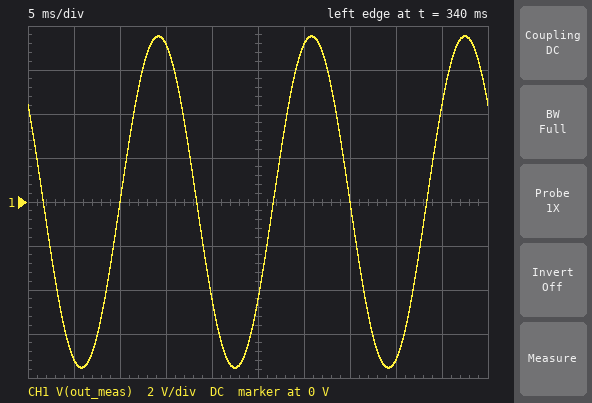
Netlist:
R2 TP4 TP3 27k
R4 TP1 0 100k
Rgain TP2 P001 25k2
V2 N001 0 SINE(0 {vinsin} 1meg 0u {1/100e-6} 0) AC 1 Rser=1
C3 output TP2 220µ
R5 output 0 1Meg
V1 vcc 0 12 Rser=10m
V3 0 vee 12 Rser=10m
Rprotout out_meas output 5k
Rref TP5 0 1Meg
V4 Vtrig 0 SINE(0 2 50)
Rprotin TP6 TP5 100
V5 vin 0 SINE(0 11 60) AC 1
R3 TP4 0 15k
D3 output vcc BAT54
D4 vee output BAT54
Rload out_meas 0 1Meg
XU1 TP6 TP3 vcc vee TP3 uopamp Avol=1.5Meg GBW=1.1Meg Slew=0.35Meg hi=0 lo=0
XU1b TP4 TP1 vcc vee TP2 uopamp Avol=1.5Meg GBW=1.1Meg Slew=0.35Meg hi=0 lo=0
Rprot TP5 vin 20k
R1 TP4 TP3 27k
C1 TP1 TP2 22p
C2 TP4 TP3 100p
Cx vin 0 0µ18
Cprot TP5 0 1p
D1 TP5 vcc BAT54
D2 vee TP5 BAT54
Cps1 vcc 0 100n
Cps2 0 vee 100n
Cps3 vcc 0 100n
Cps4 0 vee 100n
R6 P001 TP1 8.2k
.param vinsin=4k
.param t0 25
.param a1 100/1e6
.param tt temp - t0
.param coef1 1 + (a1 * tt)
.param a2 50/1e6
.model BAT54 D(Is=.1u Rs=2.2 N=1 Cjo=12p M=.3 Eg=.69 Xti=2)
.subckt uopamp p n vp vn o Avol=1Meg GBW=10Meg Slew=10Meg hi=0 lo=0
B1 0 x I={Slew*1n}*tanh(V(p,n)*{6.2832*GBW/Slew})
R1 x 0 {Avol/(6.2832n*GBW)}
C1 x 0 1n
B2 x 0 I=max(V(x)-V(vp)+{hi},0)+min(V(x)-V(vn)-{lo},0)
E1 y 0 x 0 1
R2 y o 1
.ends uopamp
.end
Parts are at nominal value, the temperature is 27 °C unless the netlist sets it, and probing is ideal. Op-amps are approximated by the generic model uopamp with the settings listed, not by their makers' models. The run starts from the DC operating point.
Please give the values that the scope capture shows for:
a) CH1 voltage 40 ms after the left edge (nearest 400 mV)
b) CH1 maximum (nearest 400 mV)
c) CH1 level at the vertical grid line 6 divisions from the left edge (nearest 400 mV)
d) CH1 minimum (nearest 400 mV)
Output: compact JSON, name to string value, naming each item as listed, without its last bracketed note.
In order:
{"CH1 voltage 40 ms after the left edge": "-7.2 V", "CH1 maximum": "7.6 V", "CH1 level at the vertical grid line 6 divisions from the left edge": "7.2 V", "CH1 minimum": "-7.6 V"}
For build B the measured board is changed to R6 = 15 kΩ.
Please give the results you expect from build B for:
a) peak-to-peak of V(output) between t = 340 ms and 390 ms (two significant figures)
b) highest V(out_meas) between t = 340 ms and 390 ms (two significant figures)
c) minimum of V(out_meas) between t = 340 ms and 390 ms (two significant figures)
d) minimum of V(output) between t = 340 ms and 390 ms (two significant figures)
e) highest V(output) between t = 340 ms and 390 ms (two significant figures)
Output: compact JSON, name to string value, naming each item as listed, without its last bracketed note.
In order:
{"peak-to-peak of V(output) between t = 340 ms and 390 ms": "16 V", "highest V(out_meas) between t = 340 ms and 390 ms": "7.9 V", "minimum of V(out_meas) between t = 340 ms and 390 ms": "-7.9 V", "minimum of V(output) between t = 340 ms and 390 ms": "-8.0 V", "highest V(output) between t = 340 ms and 390 ms": "8.0 V"}
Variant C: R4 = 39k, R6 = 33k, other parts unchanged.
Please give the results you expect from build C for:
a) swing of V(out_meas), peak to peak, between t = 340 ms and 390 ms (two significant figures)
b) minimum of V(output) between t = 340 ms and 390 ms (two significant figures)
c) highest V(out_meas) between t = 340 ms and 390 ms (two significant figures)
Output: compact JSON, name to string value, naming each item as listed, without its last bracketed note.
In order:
{"swing of V(out_meas), peak to peak, between t = 340 ms and 390 ms": "24 V", "minimum of V(output) between t = 340 ms and 390 ms": "-12 V", "highest V(out_meas) between t = 340 ms and 390 ms": "12 V"}
